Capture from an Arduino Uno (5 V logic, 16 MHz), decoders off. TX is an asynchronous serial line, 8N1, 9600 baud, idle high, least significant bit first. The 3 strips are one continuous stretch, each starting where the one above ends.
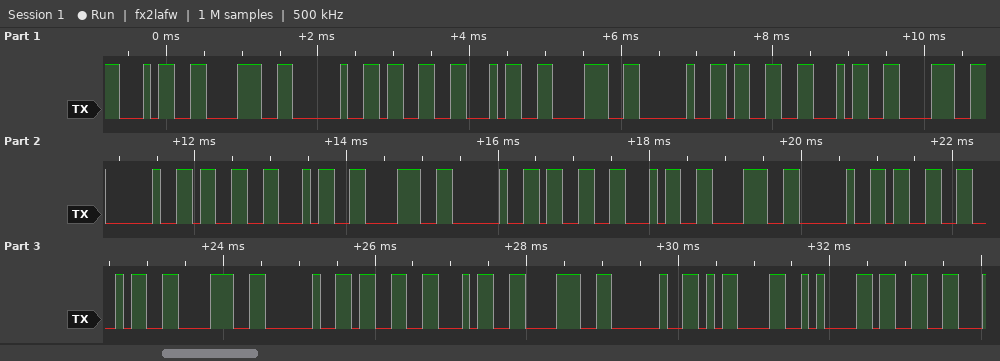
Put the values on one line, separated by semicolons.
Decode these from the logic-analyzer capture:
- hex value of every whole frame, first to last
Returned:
34 38 20 33 34 38 20 33 34 38 20 33 34 38 20 33 34 38 20 33 34 38 20 33 34 38 20 0D 0A 33
